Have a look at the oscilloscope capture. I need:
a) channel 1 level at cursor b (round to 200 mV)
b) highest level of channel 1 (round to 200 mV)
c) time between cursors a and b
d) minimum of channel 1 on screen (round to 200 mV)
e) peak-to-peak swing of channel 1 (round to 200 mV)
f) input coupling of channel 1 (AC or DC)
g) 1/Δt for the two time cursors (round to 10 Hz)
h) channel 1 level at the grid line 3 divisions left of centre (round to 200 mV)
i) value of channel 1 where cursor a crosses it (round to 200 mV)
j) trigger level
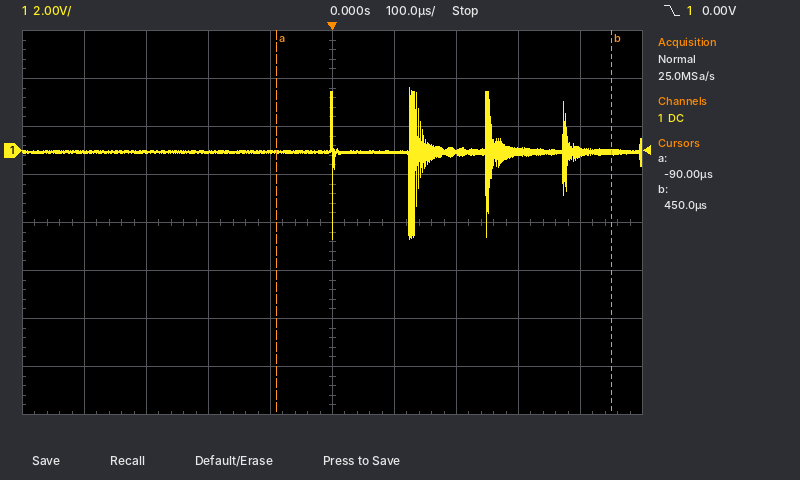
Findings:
0.0 V
2.6 V
540 µs
-3.6 V
6.2 V
DC
1.85 kHz
0.0 V
0.0 V
0.00 V
